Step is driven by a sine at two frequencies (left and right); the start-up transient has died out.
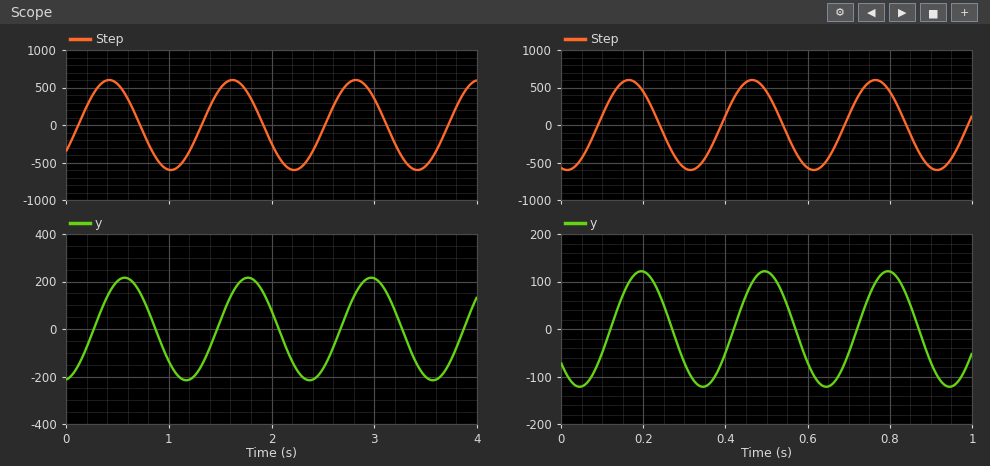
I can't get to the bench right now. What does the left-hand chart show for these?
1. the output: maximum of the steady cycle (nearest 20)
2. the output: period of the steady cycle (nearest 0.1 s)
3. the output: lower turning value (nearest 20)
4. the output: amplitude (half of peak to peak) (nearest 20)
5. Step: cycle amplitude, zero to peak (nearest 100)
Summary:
220
1.2 s
-220
220
600
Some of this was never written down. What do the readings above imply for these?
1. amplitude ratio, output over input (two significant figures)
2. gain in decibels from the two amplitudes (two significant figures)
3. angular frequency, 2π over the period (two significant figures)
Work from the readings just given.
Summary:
0.37
-8.7 dB
5.2 rad/s
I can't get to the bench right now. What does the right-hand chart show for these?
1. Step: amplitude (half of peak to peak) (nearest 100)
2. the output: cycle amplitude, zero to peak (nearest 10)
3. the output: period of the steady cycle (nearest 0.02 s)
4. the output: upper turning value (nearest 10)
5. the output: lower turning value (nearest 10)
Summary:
600
120
0.30 s
120
-120
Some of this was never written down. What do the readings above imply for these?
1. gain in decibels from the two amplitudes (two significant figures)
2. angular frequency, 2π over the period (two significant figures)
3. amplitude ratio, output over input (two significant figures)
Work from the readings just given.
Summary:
-14 dB
21 rad/s
0.20
